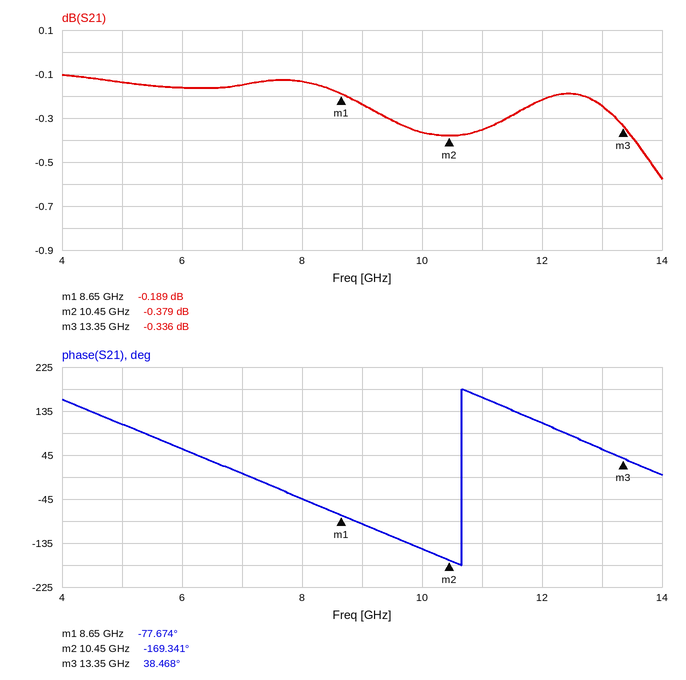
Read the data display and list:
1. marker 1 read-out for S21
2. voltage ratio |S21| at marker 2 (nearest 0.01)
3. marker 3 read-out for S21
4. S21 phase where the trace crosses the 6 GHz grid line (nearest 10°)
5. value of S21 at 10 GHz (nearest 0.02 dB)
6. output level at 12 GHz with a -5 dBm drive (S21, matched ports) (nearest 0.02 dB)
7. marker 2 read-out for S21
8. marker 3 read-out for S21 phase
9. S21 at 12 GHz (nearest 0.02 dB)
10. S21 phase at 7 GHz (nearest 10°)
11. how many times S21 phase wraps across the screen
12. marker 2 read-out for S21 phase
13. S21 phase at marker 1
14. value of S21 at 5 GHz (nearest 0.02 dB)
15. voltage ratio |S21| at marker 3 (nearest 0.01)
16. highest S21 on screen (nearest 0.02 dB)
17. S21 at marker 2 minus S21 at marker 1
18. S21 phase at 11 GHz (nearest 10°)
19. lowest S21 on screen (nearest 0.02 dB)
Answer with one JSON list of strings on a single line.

["-0.189 dB", "0.96", "-0.336 dB", "60°", "-0.36 dB", "-5.22 dBm", "-0.379 dB", "38.468°", "-0.22 dB", "10°", "1", "-169.341°", "-77.674°", "-0.14 dB", "0.96", "-0.10 dB", "-0.190 dB", "160°", "-0.58 dB"]
